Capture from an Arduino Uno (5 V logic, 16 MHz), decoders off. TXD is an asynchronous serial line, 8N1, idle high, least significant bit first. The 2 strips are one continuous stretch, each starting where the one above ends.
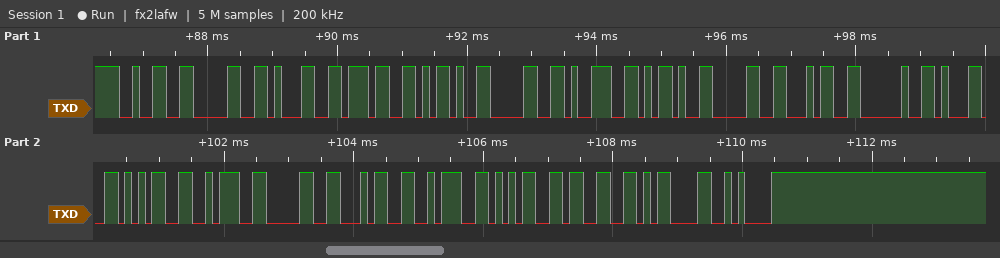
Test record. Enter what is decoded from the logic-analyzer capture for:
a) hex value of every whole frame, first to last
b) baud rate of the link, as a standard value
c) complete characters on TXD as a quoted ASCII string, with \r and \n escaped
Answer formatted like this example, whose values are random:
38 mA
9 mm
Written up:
32 30 31 37 2D 30 39 2D 30 34 20 31 35 3A 30 34 3A 35 33 0D 0A
9600 baud
"2017-09-04 15:04:53\r\n"
